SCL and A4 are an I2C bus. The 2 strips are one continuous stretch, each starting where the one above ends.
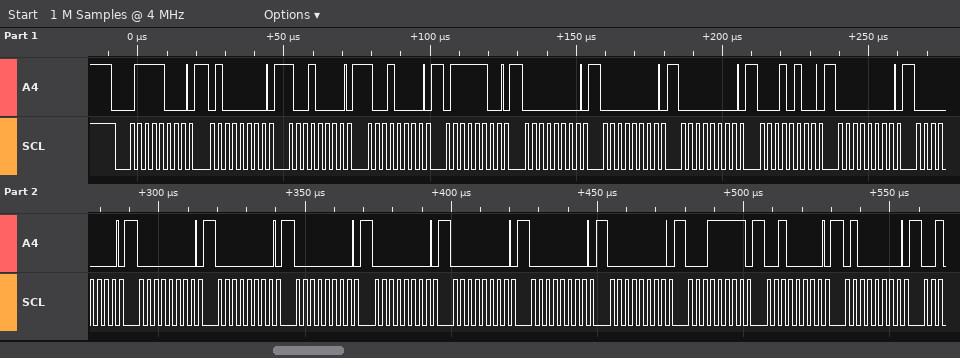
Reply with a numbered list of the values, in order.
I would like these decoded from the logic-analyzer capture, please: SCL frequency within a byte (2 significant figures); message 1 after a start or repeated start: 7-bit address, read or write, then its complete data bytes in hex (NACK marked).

1. 400 kHz
2. 0x3C write: 40 90 90 7C 00 00 00 14 00 00 00 00 00 00 00 00 00 1F 20 40
